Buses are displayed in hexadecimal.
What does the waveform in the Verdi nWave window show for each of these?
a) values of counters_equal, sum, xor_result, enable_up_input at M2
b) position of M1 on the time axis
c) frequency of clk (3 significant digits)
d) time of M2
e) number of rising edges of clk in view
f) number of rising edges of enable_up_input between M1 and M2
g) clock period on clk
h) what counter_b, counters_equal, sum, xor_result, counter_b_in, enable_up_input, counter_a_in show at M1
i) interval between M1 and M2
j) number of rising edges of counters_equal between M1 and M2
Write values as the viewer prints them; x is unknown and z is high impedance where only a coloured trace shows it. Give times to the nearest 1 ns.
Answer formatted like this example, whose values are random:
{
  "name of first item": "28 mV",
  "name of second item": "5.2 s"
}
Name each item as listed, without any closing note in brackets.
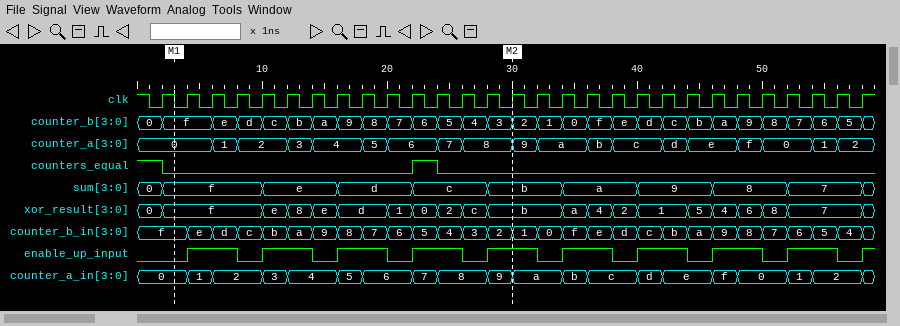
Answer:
{
  "values of counters_equal, sum, xor_result, enable_up_input at M2": "counters_equal=0, sum=b, xor_result=b, enable_up_input=1",
  "position of M1 on the time axis": "3 ns",
  "frequency of clk": "500 MHz",
  "time of M2": "30 ns",
  "number of rising edges of clk in view": "29",
  "number of rising edges of enable_up_input between M1 and M2": "5",
  "clock period on clk": "2 ns",
  "what counter_b, counters_equal, sum, xor_result, counter_b_in, enable_up_input, counter_a_in show at M1": "counter_b=f, counters_equal=0, sum=f, xor_result=f, counter_b_in=f, enable_up_input=0, counter_a_in=0",
  "interval between M1 and M2": "27 ns",
  "number of rising edges of counters_equal between M1 and M2": "1"
}
